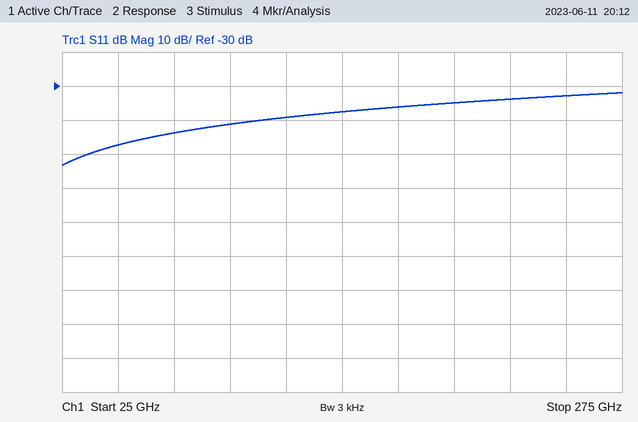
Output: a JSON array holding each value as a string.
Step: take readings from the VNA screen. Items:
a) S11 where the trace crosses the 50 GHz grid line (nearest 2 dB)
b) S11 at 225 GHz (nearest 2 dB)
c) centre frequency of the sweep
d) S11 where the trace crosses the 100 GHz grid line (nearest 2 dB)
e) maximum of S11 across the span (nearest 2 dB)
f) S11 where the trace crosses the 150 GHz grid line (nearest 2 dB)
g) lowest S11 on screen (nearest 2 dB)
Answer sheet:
["-48 dB", "-34 dB", "150 GHz", "-42 dB", "-32 dB", "-38 dB", "-54 dB"]
